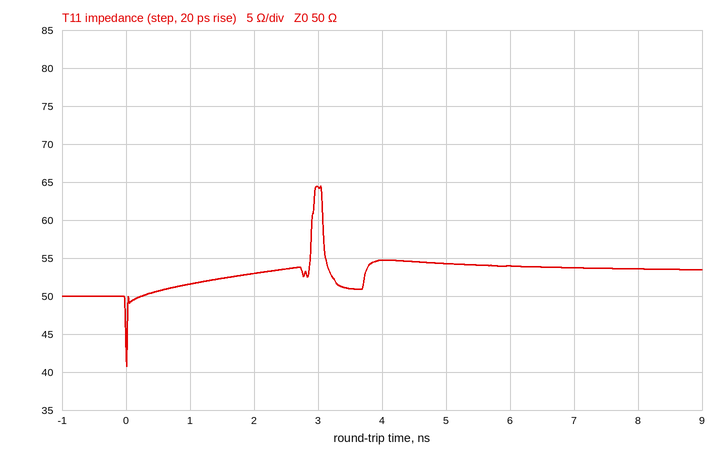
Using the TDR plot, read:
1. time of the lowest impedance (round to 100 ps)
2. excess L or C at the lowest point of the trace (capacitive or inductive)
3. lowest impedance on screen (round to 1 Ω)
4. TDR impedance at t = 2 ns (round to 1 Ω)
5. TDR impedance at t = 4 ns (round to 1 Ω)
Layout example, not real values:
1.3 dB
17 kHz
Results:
0.0 ns
capacitive
41 Ω
53 Ω
55 Ω
